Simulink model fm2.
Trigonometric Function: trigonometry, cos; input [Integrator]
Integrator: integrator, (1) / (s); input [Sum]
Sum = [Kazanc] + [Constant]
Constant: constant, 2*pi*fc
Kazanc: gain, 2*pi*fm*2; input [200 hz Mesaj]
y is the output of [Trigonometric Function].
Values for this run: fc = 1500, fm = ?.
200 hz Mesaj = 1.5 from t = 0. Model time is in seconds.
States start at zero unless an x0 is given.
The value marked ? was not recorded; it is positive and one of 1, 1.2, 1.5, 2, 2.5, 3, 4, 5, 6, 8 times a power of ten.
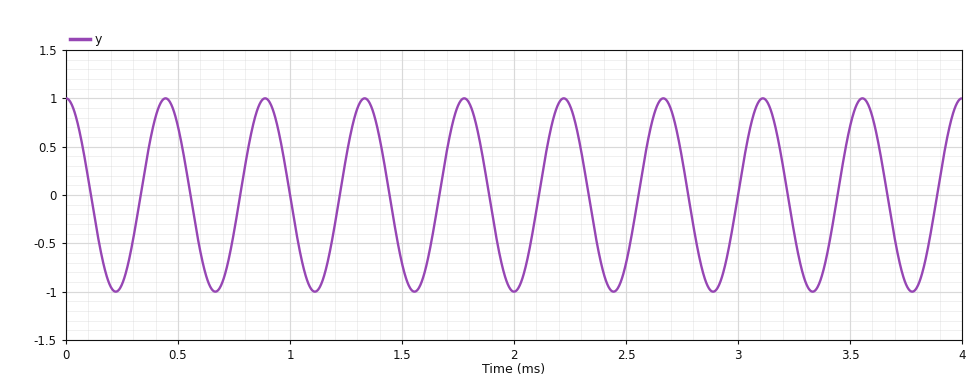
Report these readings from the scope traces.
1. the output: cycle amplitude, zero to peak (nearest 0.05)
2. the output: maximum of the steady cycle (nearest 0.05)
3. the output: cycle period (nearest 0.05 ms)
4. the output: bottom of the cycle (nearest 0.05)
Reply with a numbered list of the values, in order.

1. 1.00
2. 1.00
3. 0.45 ms
4. -1.00
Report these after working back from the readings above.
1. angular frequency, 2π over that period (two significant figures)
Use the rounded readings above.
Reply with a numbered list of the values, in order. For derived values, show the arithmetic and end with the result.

1. 2π / 0.45 = 14 rad/ms
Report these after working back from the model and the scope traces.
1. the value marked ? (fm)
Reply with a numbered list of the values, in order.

1. 250
